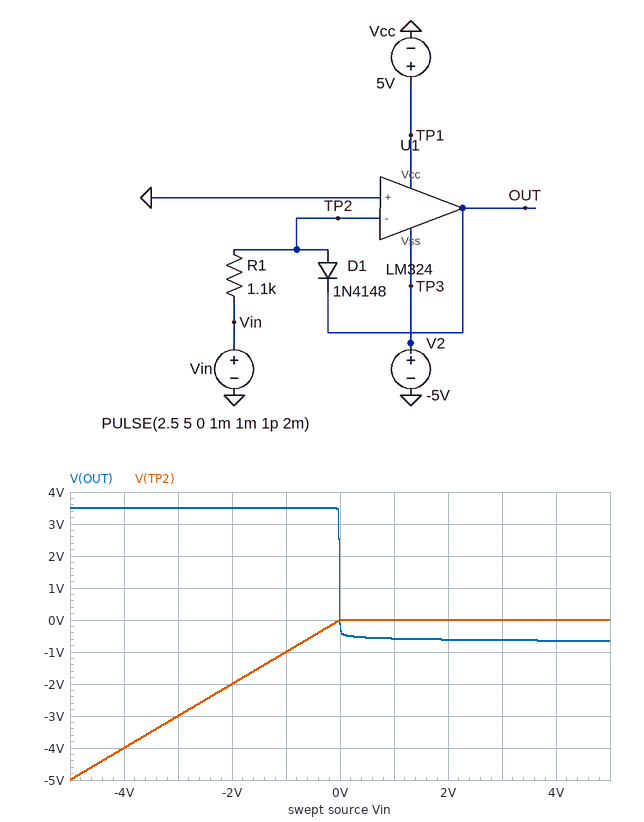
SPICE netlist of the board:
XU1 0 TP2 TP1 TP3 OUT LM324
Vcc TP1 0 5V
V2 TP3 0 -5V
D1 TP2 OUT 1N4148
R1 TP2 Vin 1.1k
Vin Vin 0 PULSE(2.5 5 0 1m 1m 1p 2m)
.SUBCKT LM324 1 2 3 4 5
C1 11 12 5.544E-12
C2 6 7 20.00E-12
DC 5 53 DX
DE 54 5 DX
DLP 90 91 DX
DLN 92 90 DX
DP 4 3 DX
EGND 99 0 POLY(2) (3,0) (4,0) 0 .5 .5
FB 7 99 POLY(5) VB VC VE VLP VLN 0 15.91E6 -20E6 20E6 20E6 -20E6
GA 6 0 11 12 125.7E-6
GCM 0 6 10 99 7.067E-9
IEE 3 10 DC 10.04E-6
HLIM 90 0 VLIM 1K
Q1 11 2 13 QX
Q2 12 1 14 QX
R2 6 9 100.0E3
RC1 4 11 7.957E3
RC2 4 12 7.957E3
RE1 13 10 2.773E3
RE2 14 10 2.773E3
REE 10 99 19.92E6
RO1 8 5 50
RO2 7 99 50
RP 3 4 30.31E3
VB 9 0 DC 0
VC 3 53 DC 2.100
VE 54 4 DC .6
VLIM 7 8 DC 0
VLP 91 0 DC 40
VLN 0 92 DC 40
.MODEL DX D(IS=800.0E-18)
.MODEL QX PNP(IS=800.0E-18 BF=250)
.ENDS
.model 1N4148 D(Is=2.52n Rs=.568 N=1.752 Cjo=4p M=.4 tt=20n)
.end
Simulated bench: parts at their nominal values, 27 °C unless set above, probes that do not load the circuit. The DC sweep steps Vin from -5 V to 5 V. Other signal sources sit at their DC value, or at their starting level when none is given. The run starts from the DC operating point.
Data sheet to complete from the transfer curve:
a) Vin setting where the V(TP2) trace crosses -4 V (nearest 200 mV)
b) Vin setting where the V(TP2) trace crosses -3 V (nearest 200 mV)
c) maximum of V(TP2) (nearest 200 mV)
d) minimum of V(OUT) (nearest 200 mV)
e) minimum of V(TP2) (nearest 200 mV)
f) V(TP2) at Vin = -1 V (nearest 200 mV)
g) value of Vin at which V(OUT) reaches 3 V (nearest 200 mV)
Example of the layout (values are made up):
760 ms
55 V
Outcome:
-4.0 V
-3.0 V
0 V
-600 mV
-5.0 V
-1.0 V
0 V
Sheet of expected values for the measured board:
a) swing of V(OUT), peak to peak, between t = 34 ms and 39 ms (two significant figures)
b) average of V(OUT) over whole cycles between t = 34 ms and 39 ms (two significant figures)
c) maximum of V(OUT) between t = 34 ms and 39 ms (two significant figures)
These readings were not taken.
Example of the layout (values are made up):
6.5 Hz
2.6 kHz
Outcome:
33 mV
-640 mV
-620 mV
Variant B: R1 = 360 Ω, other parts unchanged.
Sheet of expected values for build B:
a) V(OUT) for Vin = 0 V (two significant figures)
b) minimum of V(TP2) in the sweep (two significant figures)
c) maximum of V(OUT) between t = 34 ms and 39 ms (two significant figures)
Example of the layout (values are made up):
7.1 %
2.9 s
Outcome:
-170 mV
-5.0 V
-680 mV
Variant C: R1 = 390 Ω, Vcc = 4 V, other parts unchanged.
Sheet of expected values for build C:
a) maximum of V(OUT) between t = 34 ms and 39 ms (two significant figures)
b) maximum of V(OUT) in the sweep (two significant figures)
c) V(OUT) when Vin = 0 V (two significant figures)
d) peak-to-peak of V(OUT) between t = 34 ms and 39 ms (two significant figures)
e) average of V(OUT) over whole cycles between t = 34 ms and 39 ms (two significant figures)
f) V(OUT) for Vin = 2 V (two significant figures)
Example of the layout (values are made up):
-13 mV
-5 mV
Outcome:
-670 mV
2.5 V
-200 mV
35 mV
-690 mV
-660 mV
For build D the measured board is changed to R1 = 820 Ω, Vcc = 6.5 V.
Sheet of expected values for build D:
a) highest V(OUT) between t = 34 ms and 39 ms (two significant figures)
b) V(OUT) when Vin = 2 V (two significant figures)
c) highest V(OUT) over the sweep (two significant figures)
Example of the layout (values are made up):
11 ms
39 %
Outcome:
-640 mV
-630 mV
5.0 V
